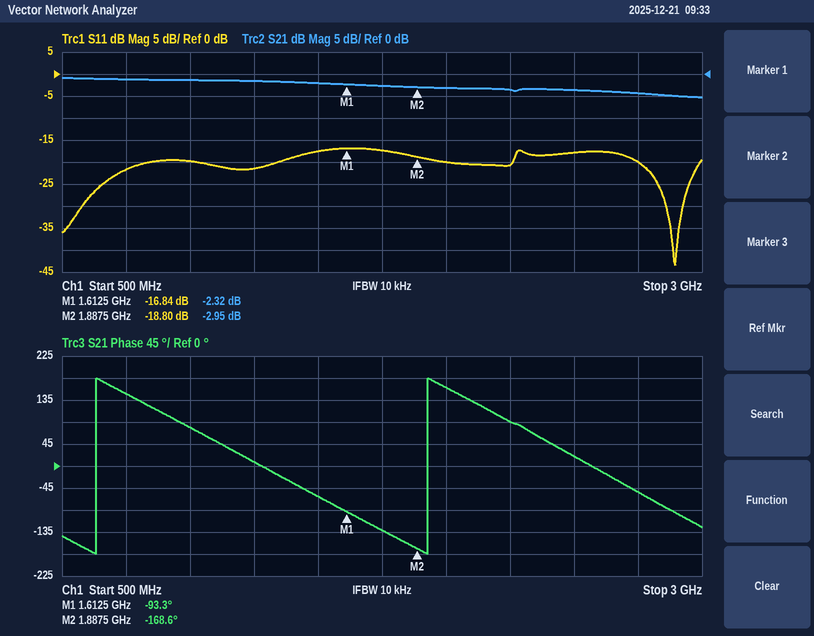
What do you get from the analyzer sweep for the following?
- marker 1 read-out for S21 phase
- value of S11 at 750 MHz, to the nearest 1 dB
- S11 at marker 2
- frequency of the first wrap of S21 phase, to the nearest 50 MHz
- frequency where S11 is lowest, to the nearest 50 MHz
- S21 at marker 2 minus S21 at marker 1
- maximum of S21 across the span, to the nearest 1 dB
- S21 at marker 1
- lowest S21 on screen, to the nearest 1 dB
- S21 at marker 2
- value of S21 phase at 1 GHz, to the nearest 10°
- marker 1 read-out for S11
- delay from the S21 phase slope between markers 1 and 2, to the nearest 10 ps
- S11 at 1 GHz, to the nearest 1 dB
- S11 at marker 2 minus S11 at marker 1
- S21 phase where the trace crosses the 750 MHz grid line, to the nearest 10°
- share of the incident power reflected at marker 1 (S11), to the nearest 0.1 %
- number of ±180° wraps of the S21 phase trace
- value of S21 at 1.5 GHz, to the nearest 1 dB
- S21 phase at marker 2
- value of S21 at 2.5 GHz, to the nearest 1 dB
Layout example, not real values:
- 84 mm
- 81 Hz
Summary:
- -93.3°
- -22 dB
- -18.80 dB
- 650 MHz
- 2.90 GHz
- -0.63 dB
- -1 dB
- -2.32 dB
- -5 dB
- -2.95 dB
- 80°
- -16.84 dB
- 760 ps
- -20 dB
- -1.96 dB
- 150°
- 2.1 %
- 2
- -2 dB
- -168.6°
- -4 dB
